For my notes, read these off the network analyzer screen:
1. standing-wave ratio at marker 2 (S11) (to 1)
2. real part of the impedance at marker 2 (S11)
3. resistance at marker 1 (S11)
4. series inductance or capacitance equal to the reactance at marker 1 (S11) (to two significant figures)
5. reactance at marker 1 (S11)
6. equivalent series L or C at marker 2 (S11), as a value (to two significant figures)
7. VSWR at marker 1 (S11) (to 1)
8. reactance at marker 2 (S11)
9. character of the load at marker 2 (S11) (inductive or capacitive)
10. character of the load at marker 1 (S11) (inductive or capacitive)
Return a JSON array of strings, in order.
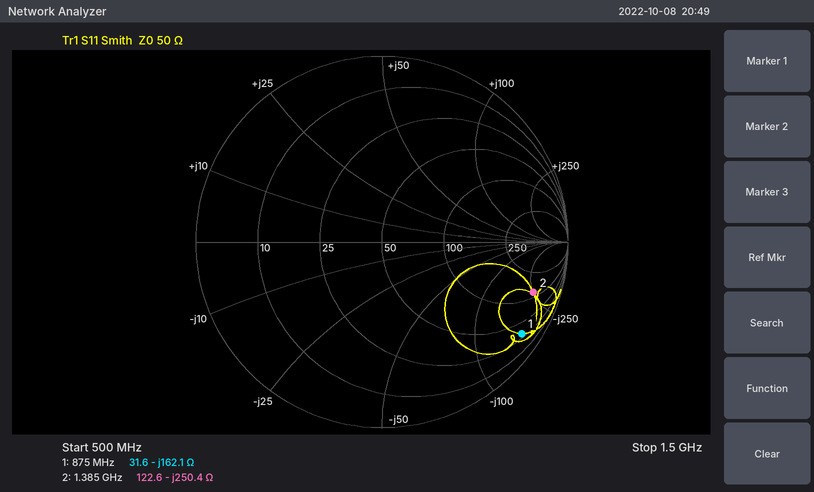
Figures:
["13", "122.6 Ω", "31.6 Ω", "1.1 pF", "-162.1 Ω", "460 fF", "19", "-250.4 Ω", "capacitive", "capacitive"]
